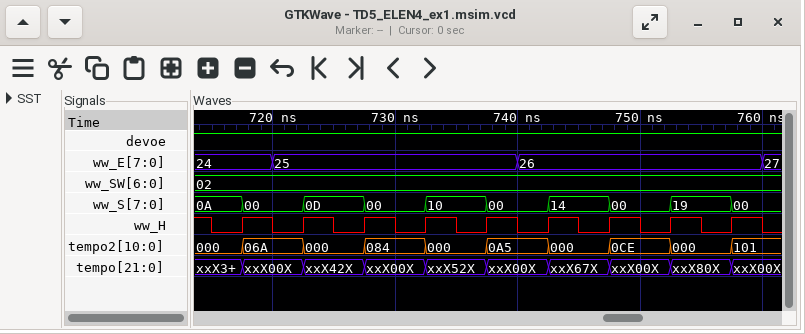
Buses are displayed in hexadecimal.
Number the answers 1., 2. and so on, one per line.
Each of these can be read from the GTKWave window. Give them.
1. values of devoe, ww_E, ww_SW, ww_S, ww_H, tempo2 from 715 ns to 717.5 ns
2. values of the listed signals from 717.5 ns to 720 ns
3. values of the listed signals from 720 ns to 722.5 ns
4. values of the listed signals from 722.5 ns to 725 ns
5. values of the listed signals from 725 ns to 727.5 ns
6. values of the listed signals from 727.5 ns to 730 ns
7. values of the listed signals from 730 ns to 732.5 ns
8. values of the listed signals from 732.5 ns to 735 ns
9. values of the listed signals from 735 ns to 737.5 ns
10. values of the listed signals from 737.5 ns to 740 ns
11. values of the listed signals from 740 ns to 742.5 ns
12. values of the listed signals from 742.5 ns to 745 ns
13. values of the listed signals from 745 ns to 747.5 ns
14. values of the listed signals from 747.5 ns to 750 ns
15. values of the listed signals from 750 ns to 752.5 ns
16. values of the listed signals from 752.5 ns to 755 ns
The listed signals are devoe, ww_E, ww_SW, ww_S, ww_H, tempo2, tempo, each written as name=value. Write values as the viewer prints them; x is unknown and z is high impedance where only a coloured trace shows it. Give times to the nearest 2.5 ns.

1. devoe=1, ww_E=24, ww_SW=02, ww_S=0A, ww_H=0, tempo2=000
2. devoe=1, ww_E=24, ww_SW=02, ww_S=00, ww_H=1, tempo2=06A, tempo=xxX00X
3. devoe=1, ww_E=25, ww_SW=02, ww_S=00, ww_H=0, tempo2=06A, tempo=xxX00X
4. devoe=1, ww_E=25, ww_SW=02, ww_S=0D, ww_H=1, tempo2=000, tempo=xxX42X
5. devoe=1, ww_E=25, ww_SW=02, ww_S=0D, ww_H=0, tempo2=000, tempo=xxX42X
6. devoe=1, ww_E=25, ww_SW=02, ww_S=00, ww_H=1, tempo2=084, tempo=xxX00X
7. devoe=1, ww_E=25, ww_SW=02, ww_S=00, ww_H=0, tempo2=084, tempo=xxX00X
8. devoe=1, ww_E=25, ww_SW=02, ww_S=10, ww_H=1, tempo2=000, tempo=xxX52X
9. devoe=1, ww_E=25, ww_SW=02, ww_S=10, ww_H=0, tempo2=000, tempo=xxX52X
10. devoe=1, ww_E=25, ww_SW=02, ww_S=00, ww_H=1, tempo2=0A5, tempo=xxX00X
11. devoe=1, ww_E=26, ww_SW=02, ww_S=00, ww_H=0, tempo2=0A5, tempo=xxX00X
12. devoe=1, ww_E=26, ww_SW=02, ww_S=14, ww_H=1, tempo2=000, tempo=xxX67X
13. devoe=1, ww_E=26, ww_SW=02, ww_S=14, ww_H=0, tempo2=000, tempo=xxX67X
14. devoe=1, ww_E=26, ww_SW=02, ww_S=00, ww_H=1, tempo2=0CE, tempo=xxX00X
15. devoe=1, ww_E=26, ww_SW=02, ww_S=00, ww_H=0, tempo2=0CE, tempo=xxX00X
16. devoe=1, ww_E=26, ww_SW=02, ww_S=19, ww_H=1, tempo2=000, tempo=xxX80X
